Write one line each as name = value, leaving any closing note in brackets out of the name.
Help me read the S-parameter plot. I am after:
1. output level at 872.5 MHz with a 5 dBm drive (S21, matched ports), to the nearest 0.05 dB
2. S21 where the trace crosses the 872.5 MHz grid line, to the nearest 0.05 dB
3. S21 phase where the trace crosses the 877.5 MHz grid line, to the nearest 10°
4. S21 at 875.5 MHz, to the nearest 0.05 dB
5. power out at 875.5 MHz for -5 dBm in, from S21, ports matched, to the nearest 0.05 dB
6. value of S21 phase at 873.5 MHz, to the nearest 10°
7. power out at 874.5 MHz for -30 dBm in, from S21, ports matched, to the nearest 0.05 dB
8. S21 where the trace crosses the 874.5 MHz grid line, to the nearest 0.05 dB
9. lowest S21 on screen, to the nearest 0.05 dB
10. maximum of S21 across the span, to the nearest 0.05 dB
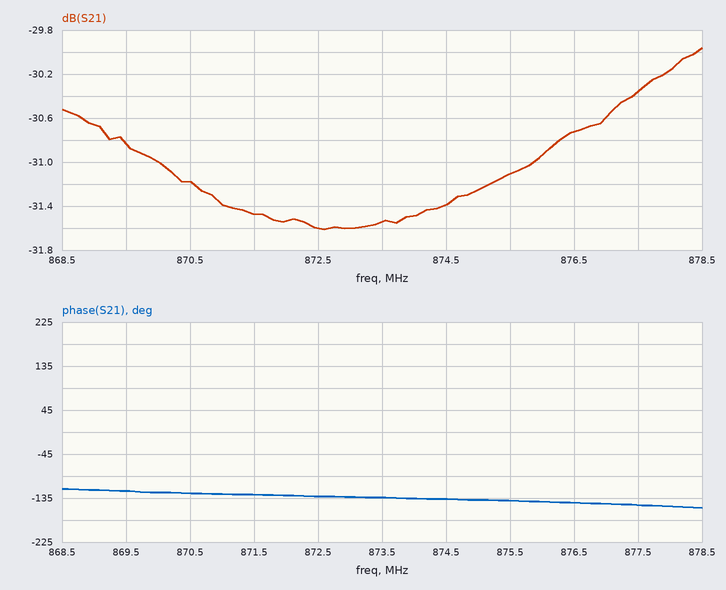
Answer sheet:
output level at 872.5 MHz with a 5 dBm drive (S21, matched ports), to the nearest 0.05 dB = -26.60 dBm
S21 where the trace crosses the 872.5 MHz grid line, to the nearest 0.05 dB = -31.60 dB
S21 phase where the trace crosses the 877.5 MHz grid line, to the nearest 10° = -150°
S21 at 875.5 MHz, to the nearest 0.05 dB = -31.10 dB
power out at 875.5 MHz for -5 dBm in, from S21, ports matched, to the nearest 0.05 dB = -36.10 dBm
value of S21 phase at 873.5 MHz, to the nearest 10° = -130°
power out at 874.5 MHz for -30 dBm in, from S21, ports matched, to the nearest 0.05 dB = -61.40 dBm
S21 where the trace crosses the 874.5 MHz grid line, to the nearest 0.05 dB = -31.40 dB
lowest S21 on screen, to the nearest 0.05 dB = -31.60 dB
maximum of S21 across the span, to the nearest 0.05 dB = -29.95 dB
